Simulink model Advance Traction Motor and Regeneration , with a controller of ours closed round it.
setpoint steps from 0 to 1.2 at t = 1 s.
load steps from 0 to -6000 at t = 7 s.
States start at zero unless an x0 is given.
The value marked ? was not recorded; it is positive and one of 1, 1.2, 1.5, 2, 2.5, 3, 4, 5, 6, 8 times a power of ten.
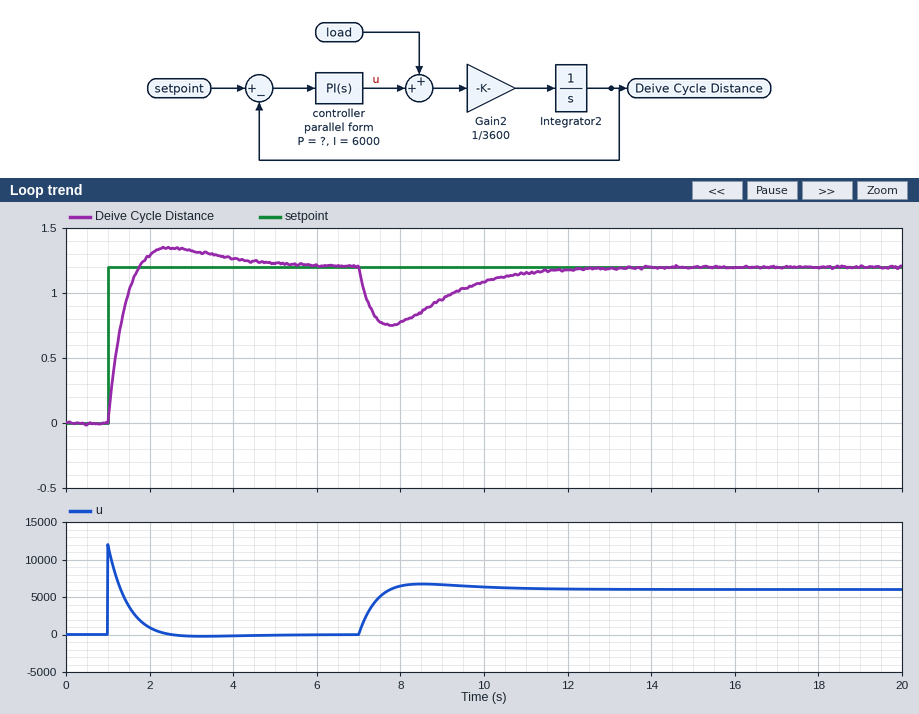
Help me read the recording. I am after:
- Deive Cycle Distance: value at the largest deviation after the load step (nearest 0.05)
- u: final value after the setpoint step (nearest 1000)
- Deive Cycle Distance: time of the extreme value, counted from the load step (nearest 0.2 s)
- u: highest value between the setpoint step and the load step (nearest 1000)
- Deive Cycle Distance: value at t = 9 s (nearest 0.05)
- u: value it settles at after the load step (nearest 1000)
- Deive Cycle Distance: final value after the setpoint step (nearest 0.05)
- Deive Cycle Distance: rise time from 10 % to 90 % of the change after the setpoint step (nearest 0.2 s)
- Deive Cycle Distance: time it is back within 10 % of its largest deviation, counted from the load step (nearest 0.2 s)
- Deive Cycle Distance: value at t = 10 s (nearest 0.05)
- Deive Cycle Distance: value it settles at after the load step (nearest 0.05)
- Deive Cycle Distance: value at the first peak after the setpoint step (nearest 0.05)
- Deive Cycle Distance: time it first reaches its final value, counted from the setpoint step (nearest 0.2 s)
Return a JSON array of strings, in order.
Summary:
["0.75", "0", "0.8 s", "12000", "0.95", "6000", "1.20", "0.6 s", "4.0 s", "1.10", "1.20", "1.35", "0.8 s"]
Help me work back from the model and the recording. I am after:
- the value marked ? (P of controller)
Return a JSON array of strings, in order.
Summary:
["10000"]
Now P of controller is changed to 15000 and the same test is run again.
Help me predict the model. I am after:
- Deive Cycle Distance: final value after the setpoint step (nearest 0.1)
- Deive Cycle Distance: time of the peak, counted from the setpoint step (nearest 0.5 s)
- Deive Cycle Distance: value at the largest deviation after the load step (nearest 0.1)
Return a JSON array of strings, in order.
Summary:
["1.2", "1.5 s", "0.9"]
